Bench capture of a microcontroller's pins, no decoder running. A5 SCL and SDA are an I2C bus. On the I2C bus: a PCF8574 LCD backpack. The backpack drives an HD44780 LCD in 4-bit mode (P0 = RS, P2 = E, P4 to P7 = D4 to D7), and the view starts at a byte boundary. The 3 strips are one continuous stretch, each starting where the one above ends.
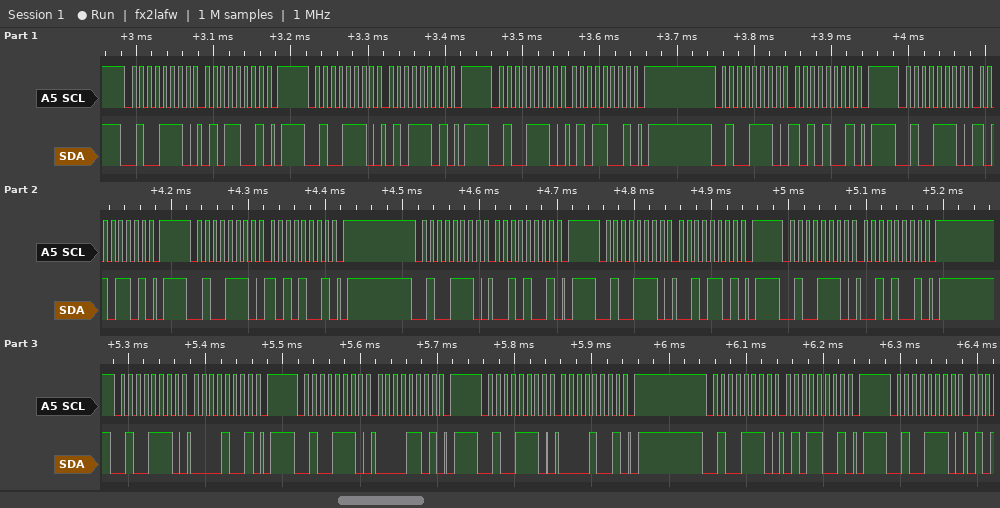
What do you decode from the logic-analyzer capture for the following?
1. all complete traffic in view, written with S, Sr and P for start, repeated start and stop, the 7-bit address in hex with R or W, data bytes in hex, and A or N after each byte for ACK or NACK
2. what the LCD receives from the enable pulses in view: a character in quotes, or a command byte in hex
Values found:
S 27W A 59 A P S 27W A 5D A P S 27W A 59 A P S 27W A A9 A P S 27W A AD A P S 27W A A9 A P S 27W A 29 A P S 27W A 2D A P S 27W A 29 A P S 27W A 09 A P S 27W A 0D A P S 27W A 09 A P S 27W A 59 A P S 27W A
'Z' ' '
